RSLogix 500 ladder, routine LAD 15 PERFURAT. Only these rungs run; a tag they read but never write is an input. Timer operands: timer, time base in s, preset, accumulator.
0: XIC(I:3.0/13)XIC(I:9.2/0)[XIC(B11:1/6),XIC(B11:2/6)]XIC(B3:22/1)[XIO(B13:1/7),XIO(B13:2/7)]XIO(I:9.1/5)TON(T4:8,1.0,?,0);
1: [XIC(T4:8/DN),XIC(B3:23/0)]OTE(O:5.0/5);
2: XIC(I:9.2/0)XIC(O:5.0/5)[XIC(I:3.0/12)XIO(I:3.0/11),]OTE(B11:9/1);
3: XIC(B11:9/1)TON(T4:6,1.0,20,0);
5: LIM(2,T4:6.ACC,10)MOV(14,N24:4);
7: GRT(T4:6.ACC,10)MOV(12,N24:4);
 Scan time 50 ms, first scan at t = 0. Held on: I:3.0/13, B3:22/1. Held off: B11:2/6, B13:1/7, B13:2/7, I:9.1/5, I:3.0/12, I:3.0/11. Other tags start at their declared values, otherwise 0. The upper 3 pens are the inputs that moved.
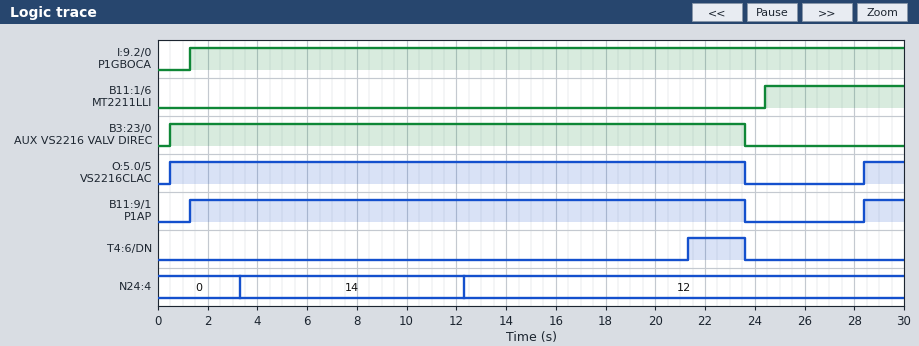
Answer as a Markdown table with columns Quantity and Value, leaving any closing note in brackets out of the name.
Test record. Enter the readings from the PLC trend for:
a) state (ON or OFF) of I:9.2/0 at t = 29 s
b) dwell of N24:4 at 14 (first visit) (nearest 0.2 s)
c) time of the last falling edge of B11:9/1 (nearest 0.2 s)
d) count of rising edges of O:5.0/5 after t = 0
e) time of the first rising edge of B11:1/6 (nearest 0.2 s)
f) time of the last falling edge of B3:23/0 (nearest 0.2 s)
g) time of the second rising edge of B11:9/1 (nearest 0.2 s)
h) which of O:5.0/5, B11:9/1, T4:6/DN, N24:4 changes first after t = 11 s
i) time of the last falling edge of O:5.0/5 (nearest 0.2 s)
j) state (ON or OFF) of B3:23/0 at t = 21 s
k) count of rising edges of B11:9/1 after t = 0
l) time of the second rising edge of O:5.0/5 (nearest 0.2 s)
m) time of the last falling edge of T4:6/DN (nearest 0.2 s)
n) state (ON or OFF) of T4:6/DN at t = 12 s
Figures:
| Quantity | Value |
|---|---|
| state (ON or OFF) of I:9.2/0 at t = 29 s | ON |
| dwell of N24:4 at 14 (first visit) | 9.0 s |
| time of the last falling edge of B11:9/1 | 23.6 s |
| count of rising edges of O:5.0/5 after t = 0 | 2 |
| time of the first rising edge of B11:1/6 | 24.4 s |
| time of the last falling edge of B3:23/0 | 23.6 s |
| time of the second rising edge of B11:9/1 | 28.4 s |
| which of O:5.0/5, B11:9/1, T4:6/DN, N24:4 changes first after t = 11 s | N24:4 |
| time of the last falling edge of O:5.0/5 | 23.6 s |
| state (ON or OFF) of B3:23/0 at t = 21 s | ON |
| count of rising edges of B11:9/1 after t = 0 | 2 |
| time of the second rising edge of O:5.0/5 | 28.4 s |
| time of the last falling edge of T4:6/DN | 23.6 s |
| state (ON or OFF) of T4:6/DN at t = 12 s | OFF |
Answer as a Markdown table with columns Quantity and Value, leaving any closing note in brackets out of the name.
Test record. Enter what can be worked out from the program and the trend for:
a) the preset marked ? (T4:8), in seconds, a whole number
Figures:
| Quantity | Value |
|---|---|
| the preset marked ? (T4:8), in seconds, a whole number | 4 s |
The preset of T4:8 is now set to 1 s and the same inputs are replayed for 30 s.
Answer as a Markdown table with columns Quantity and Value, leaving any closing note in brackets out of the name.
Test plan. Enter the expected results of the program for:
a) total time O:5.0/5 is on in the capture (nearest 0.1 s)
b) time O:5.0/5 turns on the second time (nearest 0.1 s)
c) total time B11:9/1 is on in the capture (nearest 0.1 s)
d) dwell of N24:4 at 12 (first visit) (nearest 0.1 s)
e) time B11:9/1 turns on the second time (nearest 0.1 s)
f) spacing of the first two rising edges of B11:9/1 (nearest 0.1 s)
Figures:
| Quantity | Value |
|---|---|
| total time O:5.0/5 is on in the capture | 27.7 s |
| time O:5.0/5 turns on the second time | 25.4 s |
| total time B11:9/1 is on in the capture | 26.9 s |
| dwell of N24:4 at 12 (first visit) | 15.1 s |
| time B11:9/1 turns on the second time | 25.4 s |
| spacing of the first two rising edges of B11:9/1 | 24.1 s |
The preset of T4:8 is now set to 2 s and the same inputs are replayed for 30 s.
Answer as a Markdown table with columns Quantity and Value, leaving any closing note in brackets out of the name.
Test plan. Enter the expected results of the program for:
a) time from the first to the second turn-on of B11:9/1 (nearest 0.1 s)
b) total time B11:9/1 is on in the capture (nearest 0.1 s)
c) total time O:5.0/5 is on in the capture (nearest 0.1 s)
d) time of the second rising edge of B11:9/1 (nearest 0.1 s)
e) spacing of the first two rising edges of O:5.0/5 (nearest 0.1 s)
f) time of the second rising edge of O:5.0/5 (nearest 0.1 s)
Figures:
| Quantity | Value |
|---|---|
| time from the first to the second turn-on of B11:9/1 | 25.1 s |
| total time B11:9/1 is on in the capture | 25.9 s |
| total time O:5.0/5 is on in the capture | 26.7 s |
| time of the second rising edge of B11:9/1 | 26.4 s |
| spacing of the first two rising edges of O:5.0/5 | 25.9 s |
| time of the second rising edge of O:5.0/5 | 26.4 s |
